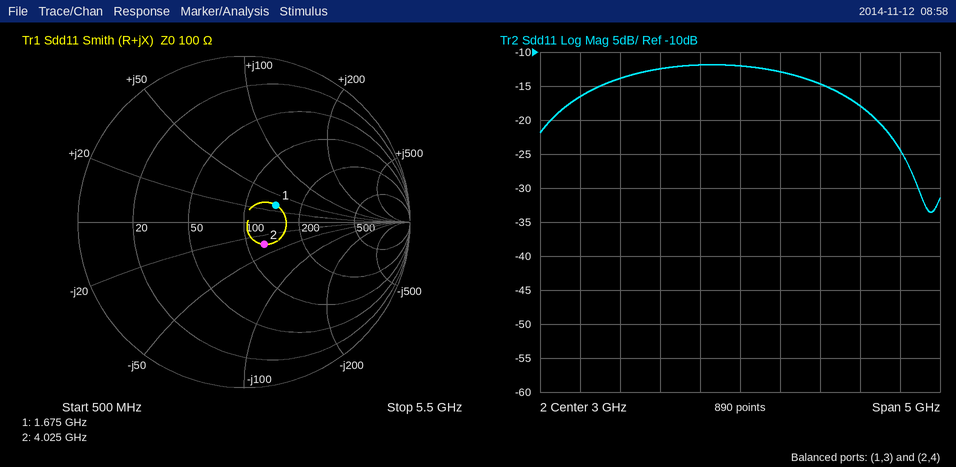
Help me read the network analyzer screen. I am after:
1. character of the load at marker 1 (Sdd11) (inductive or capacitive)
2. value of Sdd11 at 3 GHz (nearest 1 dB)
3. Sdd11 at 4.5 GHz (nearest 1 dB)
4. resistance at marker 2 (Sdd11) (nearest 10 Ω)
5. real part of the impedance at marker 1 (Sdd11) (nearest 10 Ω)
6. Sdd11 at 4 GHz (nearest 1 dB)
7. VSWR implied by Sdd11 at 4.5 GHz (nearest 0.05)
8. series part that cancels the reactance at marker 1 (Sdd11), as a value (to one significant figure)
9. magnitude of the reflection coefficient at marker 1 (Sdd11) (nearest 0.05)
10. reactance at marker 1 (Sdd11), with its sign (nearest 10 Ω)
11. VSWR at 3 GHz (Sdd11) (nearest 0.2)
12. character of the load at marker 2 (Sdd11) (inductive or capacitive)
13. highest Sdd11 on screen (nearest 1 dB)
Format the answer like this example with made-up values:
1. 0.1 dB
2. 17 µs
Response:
1. inductive
2. -12 dB
3. -18 dB
4. 120 Ω
5. 140 Ω
6. -15 dB
7. 1.30
8. 3 pF
9. 0.20
10. +30 Ω
11. 1.6
12. capacitive
13. -12 dB
